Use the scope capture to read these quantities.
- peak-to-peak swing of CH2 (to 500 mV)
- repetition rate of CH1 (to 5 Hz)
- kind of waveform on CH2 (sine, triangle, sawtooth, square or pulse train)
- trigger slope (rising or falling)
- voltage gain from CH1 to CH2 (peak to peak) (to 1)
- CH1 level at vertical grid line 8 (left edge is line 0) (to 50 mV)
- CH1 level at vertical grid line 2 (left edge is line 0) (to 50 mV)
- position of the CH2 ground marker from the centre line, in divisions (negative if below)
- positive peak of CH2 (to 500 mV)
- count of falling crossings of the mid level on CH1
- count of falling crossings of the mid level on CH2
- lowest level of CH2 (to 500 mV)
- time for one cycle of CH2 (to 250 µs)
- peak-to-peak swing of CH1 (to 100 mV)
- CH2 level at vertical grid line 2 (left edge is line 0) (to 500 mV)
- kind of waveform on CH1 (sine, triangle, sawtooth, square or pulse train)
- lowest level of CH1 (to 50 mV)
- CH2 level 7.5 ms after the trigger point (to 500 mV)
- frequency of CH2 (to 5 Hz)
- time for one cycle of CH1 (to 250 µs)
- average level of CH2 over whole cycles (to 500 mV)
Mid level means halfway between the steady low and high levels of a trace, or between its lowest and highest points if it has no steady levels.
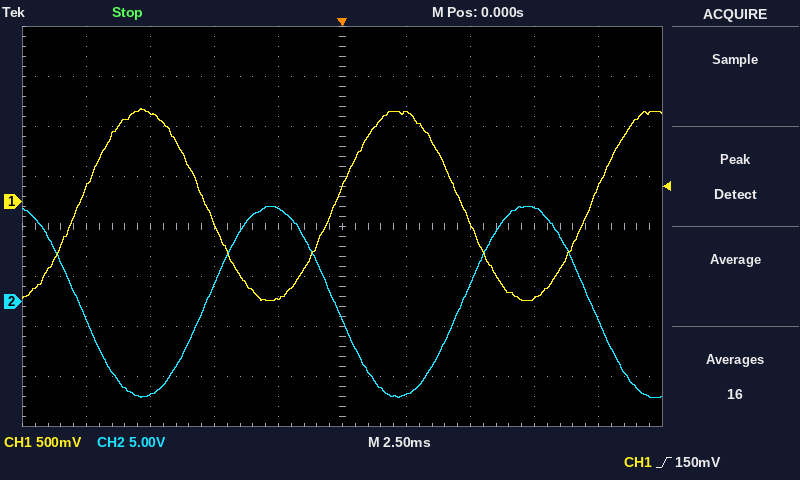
19.0 V
100 Hz
sine
rising
10
-950 mV
900 mV
-1.5 div
9.5 V
2
3
-9.5 V
10.00 ms
1.90 V
-9.5 V
sine
-1.00 V
9.5 V
100 Hz
10.00 ms
0.0 V
